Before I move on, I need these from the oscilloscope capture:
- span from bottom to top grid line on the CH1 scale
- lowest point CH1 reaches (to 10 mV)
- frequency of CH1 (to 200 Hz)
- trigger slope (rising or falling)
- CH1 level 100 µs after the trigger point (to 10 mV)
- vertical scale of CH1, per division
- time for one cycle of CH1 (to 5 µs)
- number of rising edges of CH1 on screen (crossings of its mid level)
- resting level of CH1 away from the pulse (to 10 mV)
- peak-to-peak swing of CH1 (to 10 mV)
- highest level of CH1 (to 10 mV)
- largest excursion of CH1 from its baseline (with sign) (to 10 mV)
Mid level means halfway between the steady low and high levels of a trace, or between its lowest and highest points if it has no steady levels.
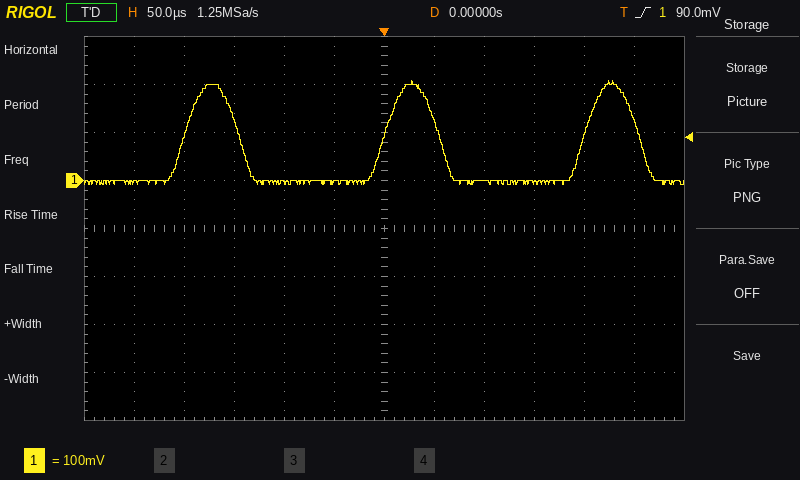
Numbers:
800 mV
-10 mV
5.0 kHz
rising
0 mV
100 mV
200 µs
3
0 mV
220 mV
210 mV
+210 mV
